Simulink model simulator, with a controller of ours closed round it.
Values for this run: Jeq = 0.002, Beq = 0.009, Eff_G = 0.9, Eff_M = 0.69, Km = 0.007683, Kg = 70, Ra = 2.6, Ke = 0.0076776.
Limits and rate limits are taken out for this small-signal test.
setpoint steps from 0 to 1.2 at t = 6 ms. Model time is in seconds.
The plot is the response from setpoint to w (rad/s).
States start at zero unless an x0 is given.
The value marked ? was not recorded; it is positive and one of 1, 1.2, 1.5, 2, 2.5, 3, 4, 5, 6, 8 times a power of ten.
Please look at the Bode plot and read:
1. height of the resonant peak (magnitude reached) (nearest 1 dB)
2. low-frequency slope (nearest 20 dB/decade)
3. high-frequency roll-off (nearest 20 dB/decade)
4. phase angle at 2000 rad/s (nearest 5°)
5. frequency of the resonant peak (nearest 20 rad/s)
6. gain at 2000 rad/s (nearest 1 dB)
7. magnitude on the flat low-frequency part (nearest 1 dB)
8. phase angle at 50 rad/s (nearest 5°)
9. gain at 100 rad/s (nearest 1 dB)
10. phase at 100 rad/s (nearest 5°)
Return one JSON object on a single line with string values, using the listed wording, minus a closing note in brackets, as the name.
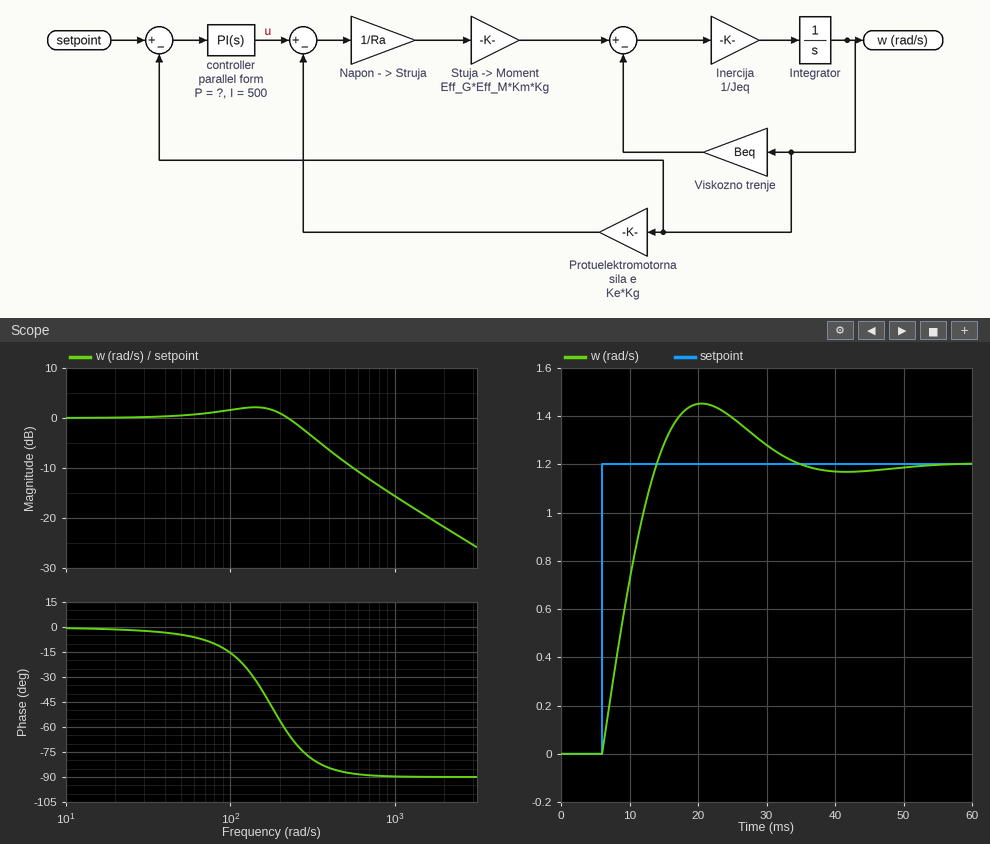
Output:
{"height of the resonant peak (magnitude reached)": "2 dB", "low-frequency slope": "0 dB/decade", "high-frequency roll-off": "-20 dB/decade", "phase angle at 2000 rad/s": "-90°", "frequency of the resonant peak": "140 rad/s", "gain at 2000 rad/s": "-22 dB", "magnitude on the flat low-frequency part": "0 dB", "phase angle at 50 rad/s": "-5°", "gain at 100 rad/s": "2 dB", "phase at 100 rad/s": "-15°"}
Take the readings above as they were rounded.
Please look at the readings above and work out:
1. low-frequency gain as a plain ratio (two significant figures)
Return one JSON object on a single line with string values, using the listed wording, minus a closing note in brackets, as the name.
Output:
{"low-frequency gain as a plain ratio": "1.0"}
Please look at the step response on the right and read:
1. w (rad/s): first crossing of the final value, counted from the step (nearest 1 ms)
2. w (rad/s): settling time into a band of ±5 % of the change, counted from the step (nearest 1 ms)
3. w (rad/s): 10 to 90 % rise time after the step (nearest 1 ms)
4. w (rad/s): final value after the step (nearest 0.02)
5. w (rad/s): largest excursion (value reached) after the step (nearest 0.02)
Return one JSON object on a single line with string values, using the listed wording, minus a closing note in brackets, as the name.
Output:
{"w (rad/s): first crossing of the final value, counted from the step": "8 ms", "w (rad/s): settling time into a band of ±5 % of the change, counted from the step": "25 ms", "w (rad/s): 10 to 90 % rise time after the step": "6 ms", "w (rad/s): final value after the step": "1.20", "w (rad/s): largest excursion (value reached) after the step": "1.46"}
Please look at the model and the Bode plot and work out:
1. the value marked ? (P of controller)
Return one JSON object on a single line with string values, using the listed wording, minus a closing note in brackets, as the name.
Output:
{"the value marked ?": "2.5"}
